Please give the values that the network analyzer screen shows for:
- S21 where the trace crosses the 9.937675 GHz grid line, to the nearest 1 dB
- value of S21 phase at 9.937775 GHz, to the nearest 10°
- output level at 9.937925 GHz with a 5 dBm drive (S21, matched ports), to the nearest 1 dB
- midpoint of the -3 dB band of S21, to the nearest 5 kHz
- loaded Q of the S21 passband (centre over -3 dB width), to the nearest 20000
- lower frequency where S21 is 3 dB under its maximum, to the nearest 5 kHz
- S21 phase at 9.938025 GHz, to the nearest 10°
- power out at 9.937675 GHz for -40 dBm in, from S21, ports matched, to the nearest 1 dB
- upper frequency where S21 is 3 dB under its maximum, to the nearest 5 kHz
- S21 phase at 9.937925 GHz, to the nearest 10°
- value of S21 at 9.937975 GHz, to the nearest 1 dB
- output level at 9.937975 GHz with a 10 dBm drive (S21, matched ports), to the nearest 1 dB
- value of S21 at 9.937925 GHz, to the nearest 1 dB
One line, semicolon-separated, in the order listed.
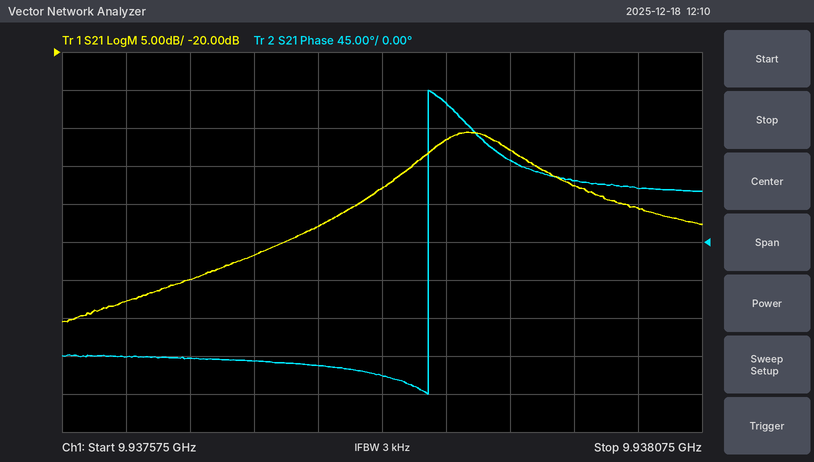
-50 dB; -150°; -28 dBm; 9.937895 GHz; 140000; 9.937860 GHz; 60°; -90 dBm; 9.937930 GHz; 100°; -38 dB; -28 dBm; -33 dB
